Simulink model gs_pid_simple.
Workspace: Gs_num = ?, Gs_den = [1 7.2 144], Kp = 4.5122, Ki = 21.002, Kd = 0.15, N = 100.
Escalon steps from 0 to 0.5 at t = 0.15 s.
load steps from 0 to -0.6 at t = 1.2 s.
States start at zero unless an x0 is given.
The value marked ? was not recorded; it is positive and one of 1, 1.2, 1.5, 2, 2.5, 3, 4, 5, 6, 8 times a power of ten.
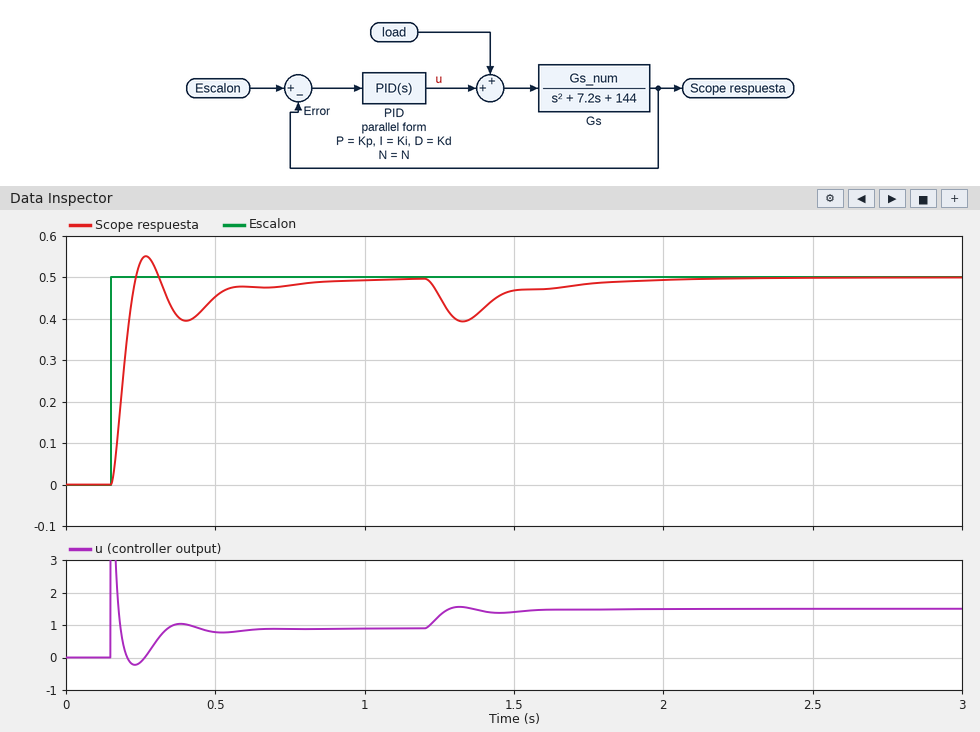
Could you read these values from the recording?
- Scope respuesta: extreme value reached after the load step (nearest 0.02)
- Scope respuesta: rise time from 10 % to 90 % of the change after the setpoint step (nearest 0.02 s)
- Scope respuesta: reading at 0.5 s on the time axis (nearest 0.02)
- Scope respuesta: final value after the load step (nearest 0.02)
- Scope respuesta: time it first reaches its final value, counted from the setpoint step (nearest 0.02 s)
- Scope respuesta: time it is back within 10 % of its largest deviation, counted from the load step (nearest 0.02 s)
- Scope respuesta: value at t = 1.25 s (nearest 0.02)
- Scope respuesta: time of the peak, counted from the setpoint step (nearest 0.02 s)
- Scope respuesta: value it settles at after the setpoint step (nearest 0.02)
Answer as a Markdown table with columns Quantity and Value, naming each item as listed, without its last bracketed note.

| Quantity | Value |
|---|---|
| Scope respuesta: extreme value reached after the load step | 0.40 |
| Scope respuesta: rise time from 10 % to 90 % of the change after the setpoint step | 0.06 s |
| Scope respuesta: reading at 0.5 s on the time axis | 0.46 |
| Scope respuesta: final value after the load step | 0.50 |
| Scope respuesta: time it first reaches its final value, counted from the setpoint step | 0.08 s |
| Scope respuesta: time it is back within 10 % of its largest deviation, counted from the load step | 0.66 s |
| Scope respuesta: value at t = 1.25 s | 0.46 |
| Scope respuesta: time of the peak, counted from the setpoint step | 0.12 s |
| Scope respuesta: value it settles at after the setpoint step | 0.50 |
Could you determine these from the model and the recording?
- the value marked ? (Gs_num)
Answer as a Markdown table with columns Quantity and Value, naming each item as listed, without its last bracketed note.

| Quantity | Value |
|---|---|
| the value marked ? | 80 |
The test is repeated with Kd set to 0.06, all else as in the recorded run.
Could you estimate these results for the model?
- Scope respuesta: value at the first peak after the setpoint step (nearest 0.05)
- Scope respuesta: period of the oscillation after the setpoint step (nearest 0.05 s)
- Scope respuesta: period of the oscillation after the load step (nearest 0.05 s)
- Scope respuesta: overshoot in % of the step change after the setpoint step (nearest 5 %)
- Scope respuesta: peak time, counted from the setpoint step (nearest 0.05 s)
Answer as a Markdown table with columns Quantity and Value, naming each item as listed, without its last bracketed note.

| Quantity | Value |
|---|---|
| Scope respuesta: value at the first peak after the setpoint step | 0.60 |
| Scope respuesta: period of the oscillation after the setpoint step | 0.30 s |
| Scope respuesta: period of the oscillation after the load step | 0.30 s |
| Scope respuesta: overshoot in % of the step change after the setpoint step | 25 % |
| Scope respuesta: peak time, counted from the setpoint step | 0.15 s |
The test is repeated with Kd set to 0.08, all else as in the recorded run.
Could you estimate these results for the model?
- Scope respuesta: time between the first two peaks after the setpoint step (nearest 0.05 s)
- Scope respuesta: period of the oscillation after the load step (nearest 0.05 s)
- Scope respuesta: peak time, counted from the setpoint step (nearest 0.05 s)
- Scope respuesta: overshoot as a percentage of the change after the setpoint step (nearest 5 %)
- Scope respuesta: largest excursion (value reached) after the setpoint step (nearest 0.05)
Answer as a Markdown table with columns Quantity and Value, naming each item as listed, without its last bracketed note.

| Quantity | Value |
|---|---|
| Scope respuesta: time between the first two peaks after the setpoint step | 0.30 s |
| Scope respuesta: period of the oscillation after the load step | 0.30 s |
| Scope respuesta: peak time, counted from the setpoint step | 0.15 s |
| Scope respuesta: overshoot as a percentage of the change after the setpoint step | 20 % |
| Scope respuesta: largest excursion (value reached) after the setpoint step | 0.60 |
